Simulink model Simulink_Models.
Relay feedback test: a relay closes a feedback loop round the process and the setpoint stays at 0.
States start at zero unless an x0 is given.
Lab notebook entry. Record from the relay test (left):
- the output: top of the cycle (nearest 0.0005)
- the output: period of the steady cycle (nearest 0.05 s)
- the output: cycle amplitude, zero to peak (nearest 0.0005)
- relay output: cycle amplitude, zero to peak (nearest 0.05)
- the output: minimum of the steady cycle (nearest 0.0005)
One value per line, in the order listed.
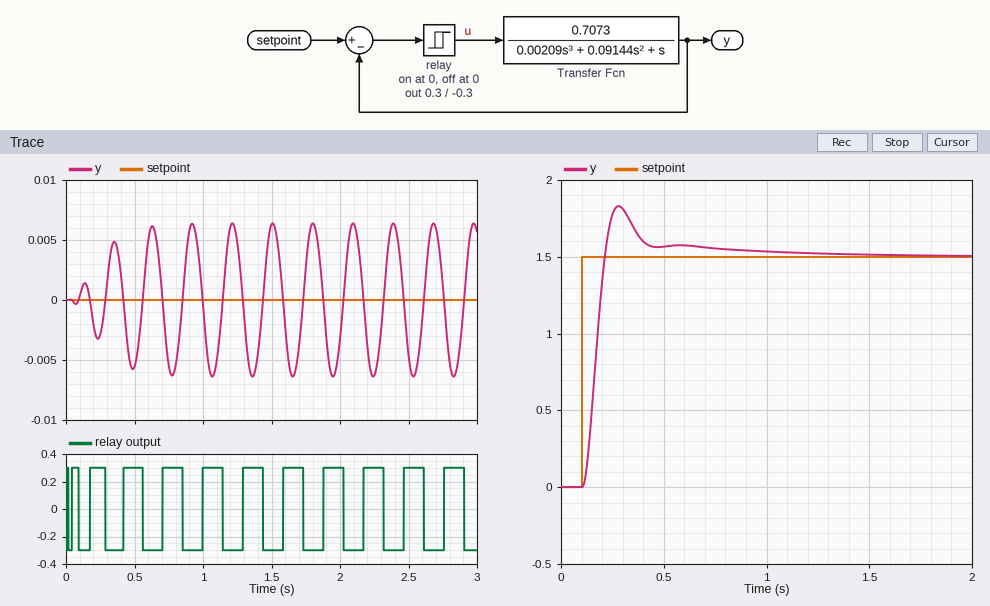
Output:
0.0065
0.30 s
0.0065
0.30
-0.0065
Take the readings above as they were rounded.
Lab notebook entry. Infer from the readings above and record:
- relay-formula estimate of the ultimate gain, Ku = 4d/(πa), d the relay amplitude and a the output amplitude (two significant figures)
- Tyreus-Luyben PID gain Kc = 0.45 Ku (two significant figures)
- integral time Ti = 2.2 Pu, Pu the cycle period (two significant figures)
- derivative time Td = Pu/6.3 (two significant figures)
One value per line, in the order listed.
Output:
59
27
0.66 s
0.048 s
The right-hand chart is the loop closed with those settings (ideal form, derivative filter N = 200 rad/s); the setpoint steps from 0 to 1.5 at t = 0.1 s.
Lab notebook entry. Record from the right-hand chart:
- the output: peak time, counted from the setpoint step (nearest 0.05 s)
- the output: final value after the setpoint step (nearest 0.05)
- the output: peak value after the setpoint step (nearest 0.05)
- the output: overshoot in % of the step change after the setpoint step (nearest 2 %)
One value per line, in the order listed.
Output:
0.20 s
1.50
1.85
22 %
